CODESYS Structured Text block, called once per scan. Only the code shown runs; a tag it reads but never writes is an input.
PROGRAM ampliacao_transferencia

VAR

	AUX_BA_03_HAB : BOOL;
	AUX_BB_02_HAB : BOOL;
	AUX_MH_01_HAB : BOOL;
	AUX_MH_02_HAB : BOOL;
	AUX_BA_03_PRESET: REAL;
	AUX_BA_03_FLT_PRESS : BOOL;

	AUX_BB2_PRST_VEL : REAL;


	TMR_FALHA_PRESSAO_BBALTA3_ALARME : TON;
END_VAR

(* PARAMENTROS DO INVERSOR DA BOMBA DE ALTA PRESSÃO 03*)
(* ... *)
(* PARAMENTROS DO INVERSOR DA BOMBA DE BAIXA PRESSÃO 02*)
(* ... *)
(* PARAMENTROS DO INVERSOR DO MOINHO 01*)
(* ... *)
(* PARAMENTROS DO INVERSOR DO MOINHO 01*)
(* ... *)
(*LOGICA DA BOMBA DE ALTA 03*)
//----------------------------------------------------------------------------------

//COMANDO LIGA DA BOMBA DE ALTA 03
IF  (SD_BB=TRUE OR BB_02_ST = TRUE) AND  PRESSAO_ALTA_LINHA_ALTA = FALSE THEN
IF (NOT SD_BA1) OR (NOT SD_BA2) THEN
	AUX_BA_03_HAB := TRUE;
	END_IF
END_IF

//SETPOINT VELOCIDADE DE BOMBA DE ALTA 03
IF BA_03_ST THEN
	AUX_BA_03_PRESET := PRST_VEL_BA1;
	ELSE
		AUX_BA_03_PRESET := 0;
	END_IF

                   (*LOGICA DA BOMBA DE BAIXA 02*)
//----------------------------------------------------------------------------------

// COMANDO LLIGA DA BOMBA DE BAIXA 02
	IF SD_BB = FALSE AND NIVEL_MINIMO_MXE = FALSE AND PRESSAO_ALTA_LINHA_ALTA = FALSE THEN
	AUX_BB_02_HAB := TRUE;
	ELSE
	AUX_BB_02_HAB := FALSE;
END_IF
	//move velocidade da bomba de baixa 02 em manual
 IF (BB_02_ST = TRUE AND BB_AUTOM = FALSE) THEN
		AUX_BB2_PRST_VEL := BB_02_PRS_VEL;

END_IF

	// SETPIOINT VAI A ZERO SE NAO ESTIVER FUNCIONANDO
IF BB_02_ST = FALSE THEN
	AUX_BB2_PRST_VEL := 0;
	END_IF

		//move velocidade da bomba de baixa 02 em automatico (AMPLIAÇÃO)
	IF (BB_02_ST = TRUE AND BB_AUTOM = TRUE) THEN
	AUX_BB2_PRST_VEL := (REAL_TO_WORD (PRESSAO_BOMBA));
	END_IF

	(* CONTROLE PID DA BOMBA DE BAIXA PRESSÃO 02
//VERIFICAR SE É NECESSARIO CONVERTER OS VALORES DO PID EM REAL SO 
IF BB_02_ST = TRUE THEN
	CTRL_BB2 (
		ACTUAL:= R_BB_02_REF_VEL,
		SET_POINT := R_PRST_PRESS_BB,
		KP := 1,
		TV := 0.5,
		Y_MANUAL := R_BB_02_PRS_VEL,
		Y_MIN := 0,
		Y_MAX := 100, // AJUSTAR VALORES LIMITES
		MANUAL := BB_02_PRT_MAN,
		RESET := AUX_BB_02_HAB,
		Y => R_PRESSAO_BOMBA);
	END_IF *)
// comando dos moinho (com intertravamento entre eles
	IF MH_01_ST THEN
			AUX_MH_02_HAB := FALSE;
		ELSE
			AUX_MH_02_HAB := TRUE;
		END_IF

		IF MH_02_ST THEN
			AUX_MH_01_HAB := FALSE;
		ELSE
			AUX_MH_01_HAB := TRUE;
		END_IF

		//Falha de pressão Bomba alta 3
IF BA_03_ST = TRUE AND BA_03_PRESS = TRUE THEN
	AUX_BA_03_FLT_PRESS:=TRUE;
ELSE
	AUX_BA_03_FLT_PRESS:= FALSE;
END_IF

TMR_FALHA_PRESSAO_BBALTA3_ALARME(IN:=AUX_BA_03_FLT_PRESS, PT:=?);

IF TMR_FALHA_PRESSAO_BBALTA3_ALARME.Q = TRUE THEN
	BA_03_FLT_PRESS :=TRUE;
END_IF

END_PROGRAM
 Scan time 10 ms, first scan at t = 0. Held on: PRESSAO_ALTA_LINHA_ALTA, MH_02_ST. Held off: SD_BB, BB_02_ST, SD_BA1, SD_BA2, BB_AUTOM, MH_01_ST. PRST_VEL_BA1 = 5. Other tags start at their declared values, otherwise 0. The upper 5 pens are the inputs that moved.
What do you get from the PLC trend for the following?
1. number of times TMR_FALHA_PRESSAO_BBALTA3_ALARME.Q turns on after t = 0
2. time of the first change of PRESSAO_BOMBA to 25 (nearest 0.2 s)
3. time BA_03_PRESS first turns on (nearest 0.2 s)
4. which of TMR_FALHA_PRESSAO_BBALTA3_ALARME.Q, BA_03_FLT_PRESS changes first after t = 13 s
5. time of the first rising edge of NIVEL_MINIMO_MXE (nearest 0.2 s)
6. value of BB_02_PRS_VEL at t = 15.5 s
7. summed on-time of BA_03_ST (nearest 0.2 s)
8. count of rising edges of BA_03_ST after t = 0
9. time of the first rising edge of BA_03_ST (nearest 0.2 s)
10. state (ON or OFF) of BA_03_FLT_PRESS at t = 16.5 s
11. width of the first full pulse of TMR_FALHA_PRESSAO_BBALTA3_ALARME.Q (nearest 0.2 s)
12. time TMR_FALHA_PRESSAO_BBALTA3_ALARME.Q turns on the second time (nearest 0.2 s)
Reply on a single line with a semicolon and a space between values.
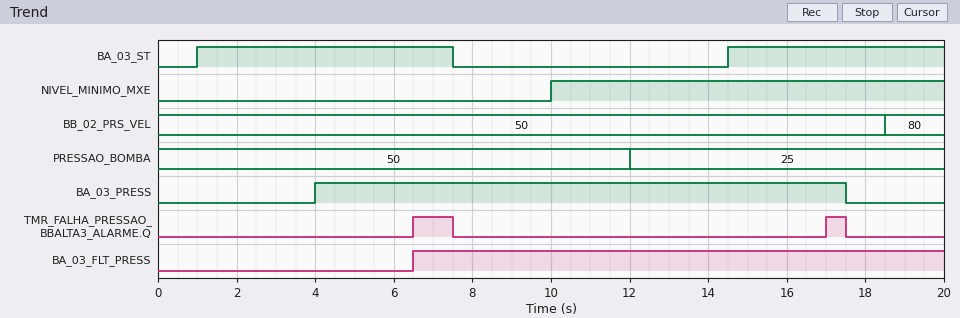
2; 12.0 s; 4.0 s; TMR_FALHA_PRESSAO_BBALTA3_ALARME.Q; 10.0 s; 50; 12.0 s; 2; 1.0 s; ON; 1.0 s; 17.0 s
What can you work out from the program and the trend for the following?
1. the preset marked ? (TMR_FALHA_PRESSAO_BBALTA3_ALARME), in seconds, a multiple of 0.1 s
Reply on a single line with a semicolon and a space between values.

2.5 s
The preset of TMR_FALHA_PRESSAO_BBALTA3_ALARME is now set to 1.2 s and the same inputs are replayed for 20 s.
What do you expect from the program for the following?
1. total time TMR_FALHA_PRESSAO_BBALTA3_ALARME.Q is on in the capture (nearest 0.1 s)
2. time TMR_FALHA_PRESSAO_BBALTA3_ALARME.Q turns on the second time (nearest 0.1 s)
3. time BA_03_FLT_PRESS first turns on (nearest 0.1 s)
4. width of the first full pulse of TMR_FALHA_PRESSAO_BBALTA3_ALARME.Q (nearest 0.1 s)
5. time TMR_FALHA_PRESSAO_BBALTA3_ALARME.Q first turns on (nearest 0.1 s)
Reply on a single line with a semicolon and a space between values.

4.1 s; 15.7 s; 5.2 s; 2.3 s; 5.2 s
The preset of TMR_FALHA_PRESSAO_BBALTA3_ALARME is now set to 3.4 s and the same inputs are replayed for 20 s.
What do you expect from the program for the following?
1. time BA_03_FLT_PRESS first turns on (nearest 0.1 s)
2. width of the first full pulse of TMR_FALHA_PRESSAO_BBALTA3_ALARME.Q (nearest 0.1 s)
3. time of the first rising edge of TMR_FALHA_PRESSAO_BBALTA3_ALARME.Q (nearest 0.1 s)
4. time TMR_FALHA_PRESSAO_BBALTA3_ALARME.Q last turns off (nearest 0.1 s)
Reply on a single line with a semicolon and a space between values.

7.4 s; 0.1 s; 7.4 s; 7.5 s
